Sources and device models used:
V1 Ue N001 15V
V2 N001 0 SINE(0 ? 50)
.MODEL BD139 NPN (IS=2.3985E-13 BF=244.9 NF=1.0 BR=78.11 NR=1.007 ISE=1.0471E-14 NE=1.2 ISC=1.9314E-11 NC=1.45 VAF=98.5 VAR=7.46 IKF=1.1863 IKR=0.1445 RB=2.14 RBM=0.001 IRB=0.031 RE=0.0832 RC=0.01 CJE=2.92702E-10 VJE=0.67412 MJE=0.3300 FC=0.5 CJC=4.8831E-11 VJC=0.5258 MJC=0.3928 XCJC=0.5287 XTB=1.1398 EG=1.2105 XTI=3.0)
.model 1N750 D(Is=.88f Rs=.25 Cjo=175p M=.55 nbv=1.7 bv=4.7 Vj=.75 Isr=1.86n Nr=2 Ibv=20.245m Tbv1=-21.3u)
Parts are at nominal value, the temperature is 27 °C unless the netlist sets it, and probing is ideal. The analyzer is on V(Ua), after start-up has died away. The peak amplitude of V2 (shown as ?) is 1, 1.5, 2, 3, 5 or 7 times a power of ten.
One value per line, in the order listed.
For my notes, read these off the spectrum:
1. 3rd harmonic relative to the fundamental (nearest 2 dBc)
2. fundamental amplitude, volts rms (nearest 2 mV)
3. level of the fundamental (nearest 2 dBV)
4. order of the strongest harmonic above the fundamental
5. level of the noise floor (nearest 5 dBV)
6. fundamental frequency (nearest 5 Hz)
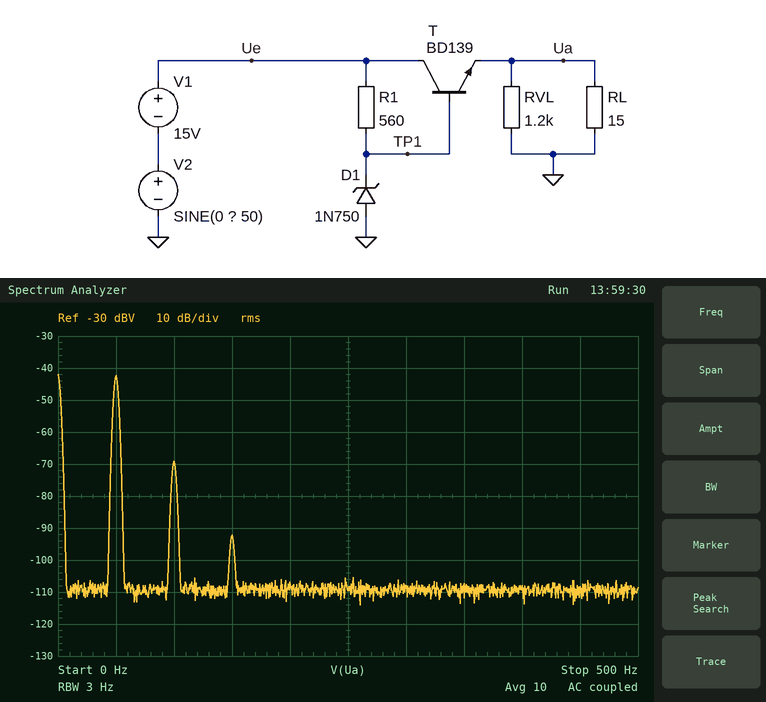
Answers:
-50 dBc
8 mV
-42 dBV
2
-110 dBV
50 Hz
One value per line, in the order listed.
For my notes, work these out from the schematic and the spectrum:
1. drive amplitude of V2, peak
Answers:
2 V
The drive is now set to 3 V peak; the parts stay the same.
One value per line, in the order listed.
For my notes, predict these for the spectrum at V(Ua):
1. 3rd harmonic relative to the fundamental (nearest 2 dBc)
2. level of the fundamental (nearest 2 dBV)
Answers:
-42 dBc
-38 dBV
